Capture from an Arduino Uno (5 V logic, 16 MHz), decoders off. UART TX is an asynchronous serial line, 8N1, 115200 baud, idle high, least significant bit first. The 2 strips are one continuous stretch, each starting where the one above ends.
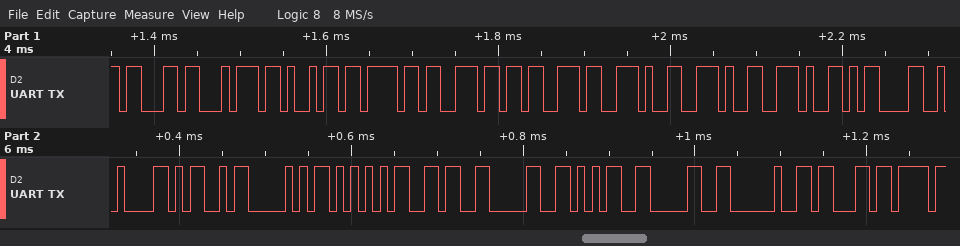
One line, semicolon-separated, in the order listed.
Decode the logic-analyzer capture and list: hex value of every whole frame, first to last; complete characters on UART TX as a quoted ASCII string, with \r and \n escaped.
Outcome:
63 74 69 6F 6E 73 2E 2E 2E 0D 0A 4D 50 55 36 30 35 30 20 63; "ctions...\r\nMPU6050 c"
